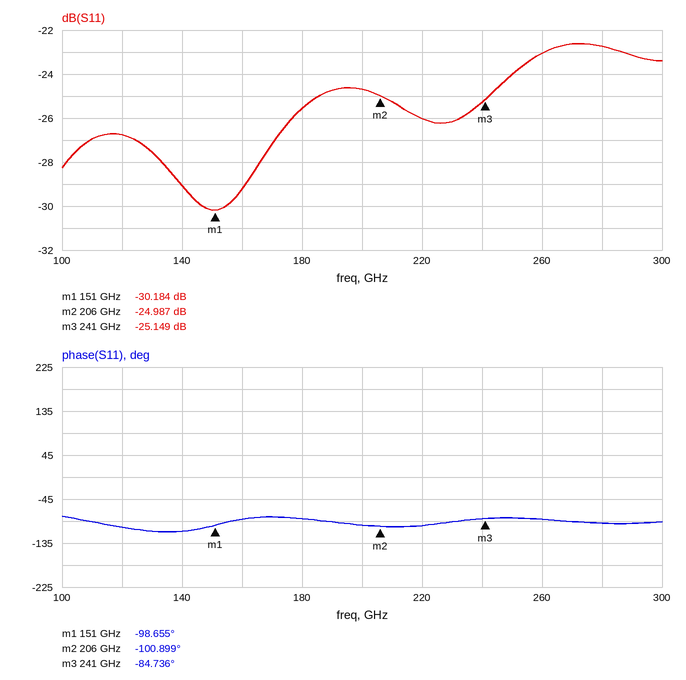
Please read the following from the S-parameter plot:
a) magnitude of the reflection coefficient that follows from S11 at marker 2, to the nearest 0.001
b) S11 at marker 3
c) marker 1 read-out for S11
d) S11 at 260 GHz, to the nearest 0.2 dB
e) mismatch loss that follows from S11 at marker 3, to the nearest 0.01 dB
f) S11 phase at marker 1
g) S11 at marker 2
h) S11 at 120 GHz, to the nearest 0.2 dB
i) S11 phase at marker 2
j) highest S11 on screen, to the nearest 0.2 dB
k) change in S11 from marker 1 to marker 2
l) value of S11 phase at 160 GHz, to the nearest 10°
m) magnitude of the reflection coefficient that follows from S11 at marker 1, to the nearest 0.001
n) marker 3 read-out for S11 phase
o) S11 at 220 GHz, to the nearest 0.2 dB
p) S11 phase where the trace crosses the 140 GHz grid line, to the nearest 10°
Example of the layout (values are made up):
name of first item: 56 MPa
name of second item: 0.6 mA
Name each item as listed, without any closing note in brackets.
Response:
magnitude of the reflection coefficient that follows from S11 at marker 2, to the nearest 0.001: 0.056
S11 at marker 3: -25.149 dB
marker 1 read-out for S11: -30.184 dB
S11 at 260 GHz, to the nearest 0.2 dB: -23.0 dB
mismatch loss that follows from S11 at marker 3, to the nearest 0.01 dB: 0.01 dB
S11 phase at marker 1: -98.655°
S11 at marker 2: -24.987 dB
S11 at 120 GHz, to the nearest 0.2 dB: -26.8 dB
S11 phase at marker 2: -100.899°
highest S11 on screen, to the nearest 0.2 dB: -22.6 dB
change in S11 from marker 1 to marker 2: 5.197 dB
value of S11 phase at 160 GHz, to the nearest 10°: -90°
magnitude of the reflection coefficient that follows from S11 at marker 1, to the nearest 0.001: 0.031
marker 3 read-out for S11 phase: -84.736°
S11 at 220 GHz, to the nearest 0.2 dB: -26.0 dB
S11 phase where the trace crosses the 140 GHz grid line, to the nearest 10°: -110°
